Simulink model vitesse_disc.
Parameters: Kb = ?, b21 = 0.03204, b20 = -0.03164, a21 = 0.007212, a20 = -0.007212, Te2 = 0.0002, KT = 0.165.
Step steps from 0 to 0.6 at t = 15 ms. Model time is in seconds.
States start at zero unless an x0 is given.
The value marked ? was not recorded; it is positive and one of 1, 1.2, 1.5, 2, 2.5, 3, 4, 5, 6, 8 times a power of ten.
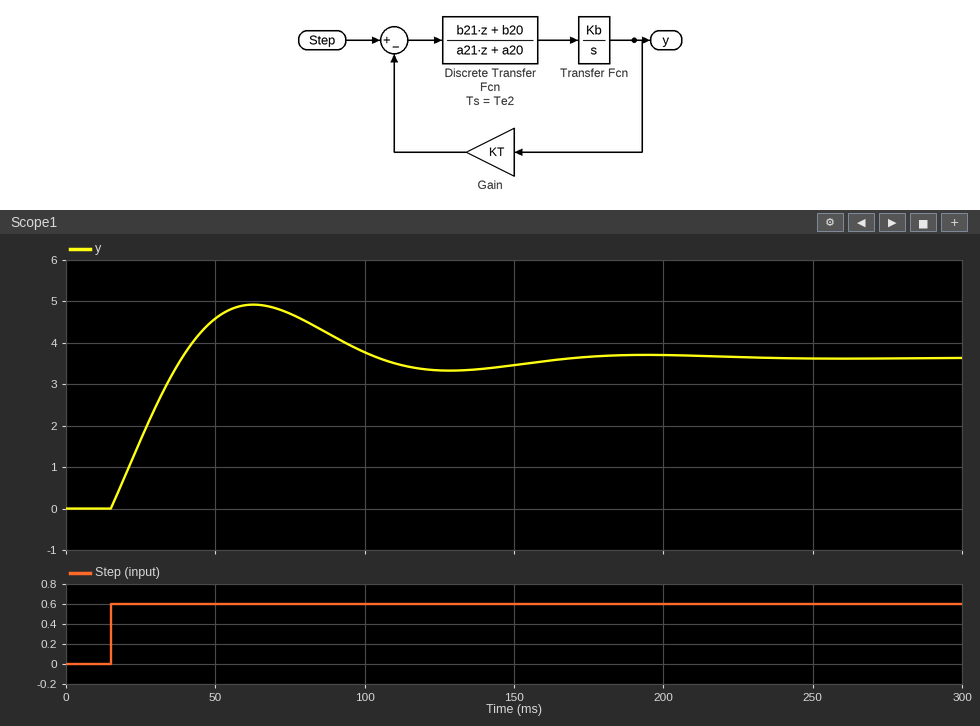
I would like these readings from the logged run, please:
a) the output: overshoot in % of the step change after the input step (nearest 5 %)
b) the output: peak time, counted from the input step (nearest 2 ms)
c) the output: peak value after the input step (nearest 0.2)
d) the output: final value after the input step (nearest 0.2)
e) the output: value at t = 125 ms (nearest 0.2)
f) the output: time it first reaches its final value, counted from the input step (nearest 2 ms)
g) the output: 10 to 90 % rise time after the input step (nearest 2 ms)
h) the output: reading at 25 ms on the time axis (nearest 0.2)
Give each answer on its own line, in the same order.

35 %
48 ms
5.0
3.6
3.4
24 ms
18 ms
1.6
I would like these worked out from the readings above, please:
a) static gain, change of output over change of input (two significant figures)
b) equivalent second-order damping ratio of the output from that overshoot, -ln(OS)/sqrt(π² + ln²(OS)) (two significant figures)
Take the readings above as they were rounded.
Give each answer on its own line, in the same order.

6.0
0.32
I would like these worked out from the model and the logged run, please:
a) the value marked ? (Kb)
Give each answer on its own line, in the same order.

60
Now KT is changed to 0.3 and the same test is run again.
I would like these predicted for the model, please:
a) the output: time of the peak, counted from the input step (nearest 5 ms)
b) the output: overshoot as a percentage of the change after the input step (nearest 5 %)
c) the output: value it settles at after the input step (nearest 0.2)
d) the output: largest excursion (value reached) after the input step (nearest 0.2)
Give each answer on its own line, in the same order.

35 ms
25 %
2.0
2.6
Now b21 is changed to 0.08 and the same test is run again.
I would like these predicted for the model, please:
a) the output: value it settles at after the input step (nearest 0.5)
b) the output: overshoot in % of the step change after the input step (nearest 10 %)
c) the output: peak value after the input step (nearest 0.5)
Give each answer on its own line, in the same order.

3.5
90 %
7.0
